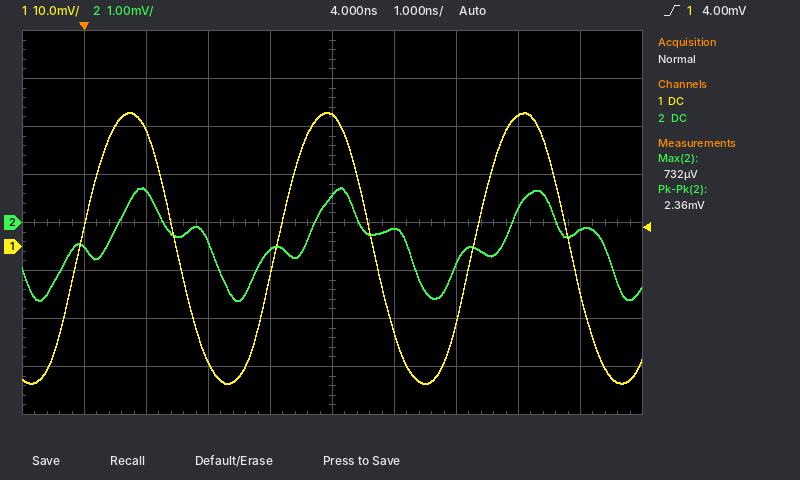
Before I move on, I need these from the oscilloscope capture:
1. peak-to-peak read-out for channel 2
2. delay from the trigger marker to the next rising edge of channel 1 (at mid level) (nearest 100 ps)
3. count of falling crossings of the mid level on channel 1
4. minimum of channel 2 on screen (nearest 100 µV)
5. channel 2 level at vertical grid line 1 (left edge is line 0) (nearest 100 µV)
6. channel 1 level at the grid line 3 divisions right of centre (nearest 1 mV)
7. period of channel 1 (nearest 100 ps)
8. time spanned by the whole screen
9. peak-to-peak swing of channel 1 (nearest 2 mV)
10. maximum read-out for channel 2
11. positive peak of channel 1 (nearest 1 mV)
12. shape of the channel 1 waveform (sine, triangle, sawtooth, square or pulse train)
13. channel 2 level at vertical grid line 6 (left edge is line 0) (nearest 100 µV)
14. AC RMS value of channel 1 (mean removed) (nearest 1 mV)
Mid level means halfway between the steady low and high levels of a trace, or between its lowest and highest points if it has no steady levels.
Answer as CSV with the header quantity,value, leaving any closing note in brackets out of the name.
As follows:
quantity,value
peak-to-peak read-out for channel 2,2.36 mV
delay from the trigger marker to the next rising edge of channel 1 (at mid level),3.1 ns
count of falling crossings of the mid level on channel 1,3
minimum of channel 2 on screen,-1.6 mV
channel 2 level at vertical grid line 1 (left edge is line 0),-500 µV
channel 1 level at the grid line 3 divisions right of centre,27 mV
period of channel 1,3.2 ns
time spanned by the whole screen,10 ns
peak-to-peak swing of channel 1,56 mV
maximum read-out for channel 2,732 µV
positive peak of channel 1,28 mV
shape of the channel 1 waveform,sine
channel 2 level at vertical grid line 6 (left edge is line 0),-100 µV
AC RMS value of channel 1 (mean removed),20 mV
